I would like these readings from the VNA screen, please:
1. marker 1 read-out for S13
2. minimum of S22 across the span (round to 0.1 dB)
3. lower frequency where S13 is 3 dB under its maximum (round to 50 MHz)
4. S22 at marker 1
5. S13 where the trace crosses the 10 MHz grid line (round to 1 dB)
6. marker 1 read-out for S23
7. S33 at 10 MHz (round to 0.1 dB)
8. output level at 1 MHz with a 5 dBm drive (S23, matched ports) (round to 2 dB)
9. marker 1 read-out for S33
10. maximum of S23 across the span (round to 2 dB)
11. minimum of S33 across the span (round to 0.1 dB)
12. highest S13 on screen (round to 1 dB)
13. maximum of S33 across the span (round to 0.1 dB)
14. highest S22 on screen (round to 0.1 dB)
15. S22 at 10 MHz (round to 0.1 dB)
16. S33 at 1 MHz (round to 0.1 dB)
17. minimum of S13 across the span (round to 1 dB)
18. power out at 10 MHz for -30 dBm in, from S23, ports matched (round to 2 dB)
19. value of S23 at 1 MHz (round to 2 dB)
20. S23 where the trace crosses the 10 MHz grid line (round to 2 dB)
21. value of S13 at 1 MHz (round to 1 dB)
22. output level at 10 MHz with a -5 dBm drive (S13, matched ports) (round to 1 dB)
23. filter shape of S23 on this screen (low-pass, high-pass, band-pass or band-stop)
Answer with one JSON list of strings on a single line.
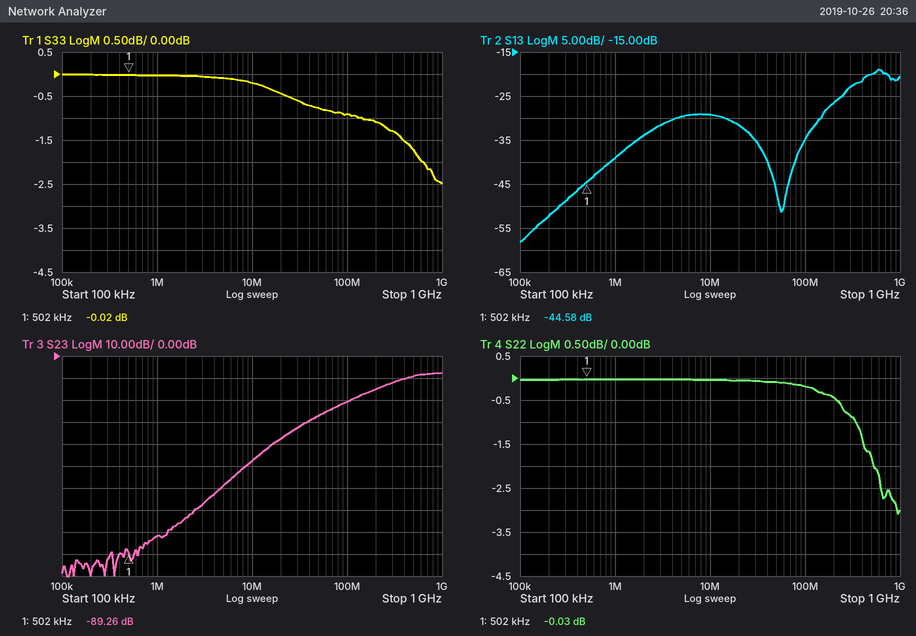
["-44.58 dB", "-3.1 dB", "350 MHz", "-0.03 dB", "-29 dB", "-89.26 dB", "-0.2 dB", "-76 dBm", "-0.02 dB", "-8 dB", "-2.5 dB", "-19 dB", "0.0 dB", "0.0 dB", "0.0 dB", "0.0 dB", "-58 dB", "-78 dBm", "-82 dB", "-48 dB", "-39 dB", "-34 dBm", "high-pass"]
